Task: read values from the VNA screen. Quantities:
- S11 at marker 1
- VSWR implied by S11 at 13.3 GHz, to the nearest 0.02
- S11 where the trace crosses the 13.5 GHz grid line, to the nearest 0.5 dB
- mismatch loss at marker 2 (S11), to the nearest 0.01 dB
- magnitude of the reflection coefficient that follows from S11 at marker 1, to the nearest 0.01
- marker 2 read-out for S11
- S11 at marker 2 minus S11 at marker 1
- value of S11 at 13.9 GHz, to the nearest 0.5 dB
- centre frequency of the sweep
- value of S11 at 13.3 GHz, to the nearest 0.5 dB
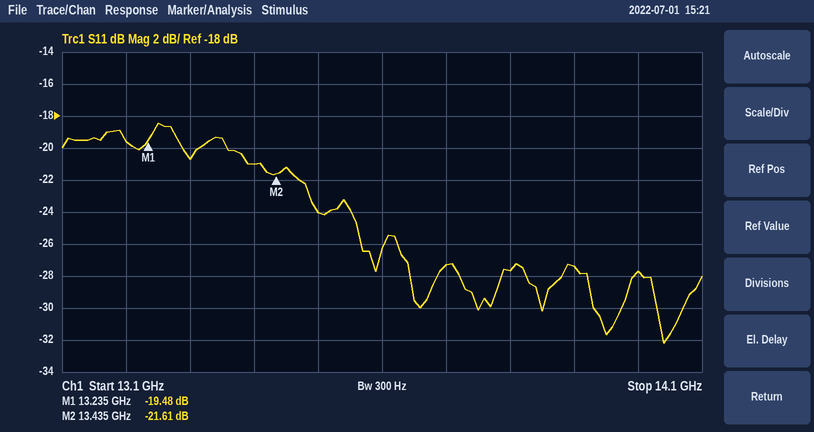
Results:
-19.48 dB
1.20
-24.0 dB
0.03 dB
0.11
-21.61 dB
-2.13 dB
-27.5 dB
13.6 GHz
-20.5 dB
